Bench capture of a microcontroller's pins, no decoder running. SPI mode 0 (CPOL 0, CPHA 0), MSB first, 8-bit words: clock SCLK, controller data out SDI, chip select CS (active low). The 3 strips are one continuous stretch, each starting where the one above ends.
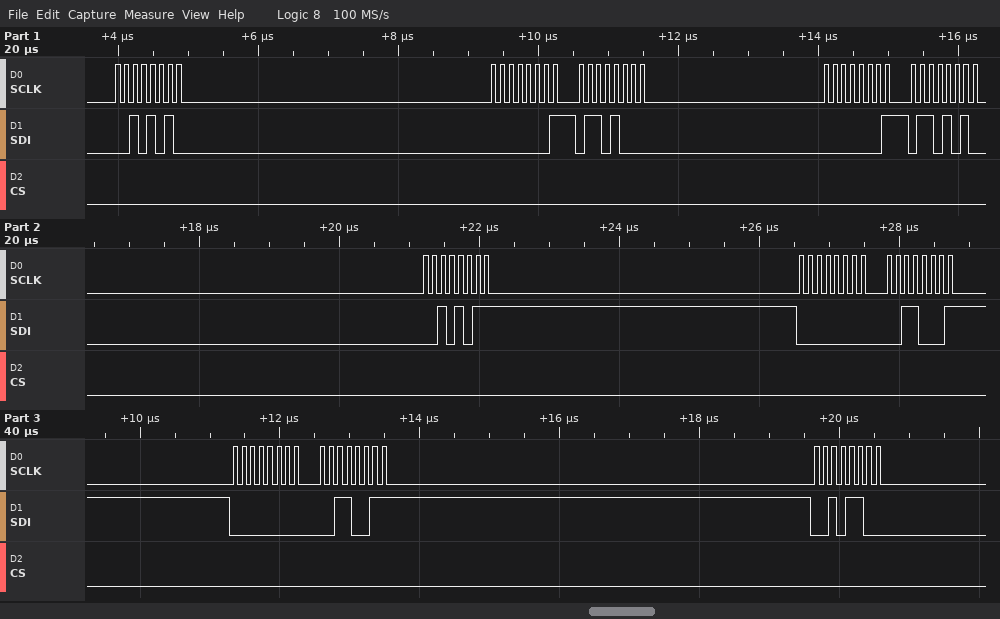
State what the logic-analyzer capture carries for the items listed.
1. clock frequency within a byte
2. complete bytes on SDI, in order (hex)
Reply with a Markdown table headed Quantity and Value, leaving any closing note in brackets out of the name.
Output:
| Quantity | Value |
|---|---|
| clock frequency within a byte | 8 MHz |
| complete bytes on SDI, in order | 2A 01 68 01 6A 2B 00 31 00 33 2C |
